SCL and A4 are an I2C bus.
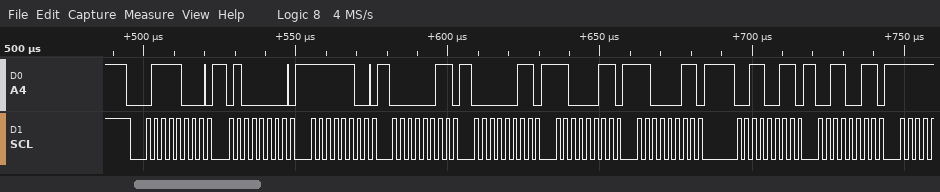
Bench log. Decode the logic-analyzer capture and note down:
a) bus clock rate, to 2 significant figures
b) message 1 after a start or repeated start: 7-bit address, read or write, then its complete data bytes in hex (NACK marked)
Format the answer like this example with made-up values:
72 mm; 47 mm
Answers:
400 kHz; 0x3C write: 40 FC 03 03 C3 C3 33 33
